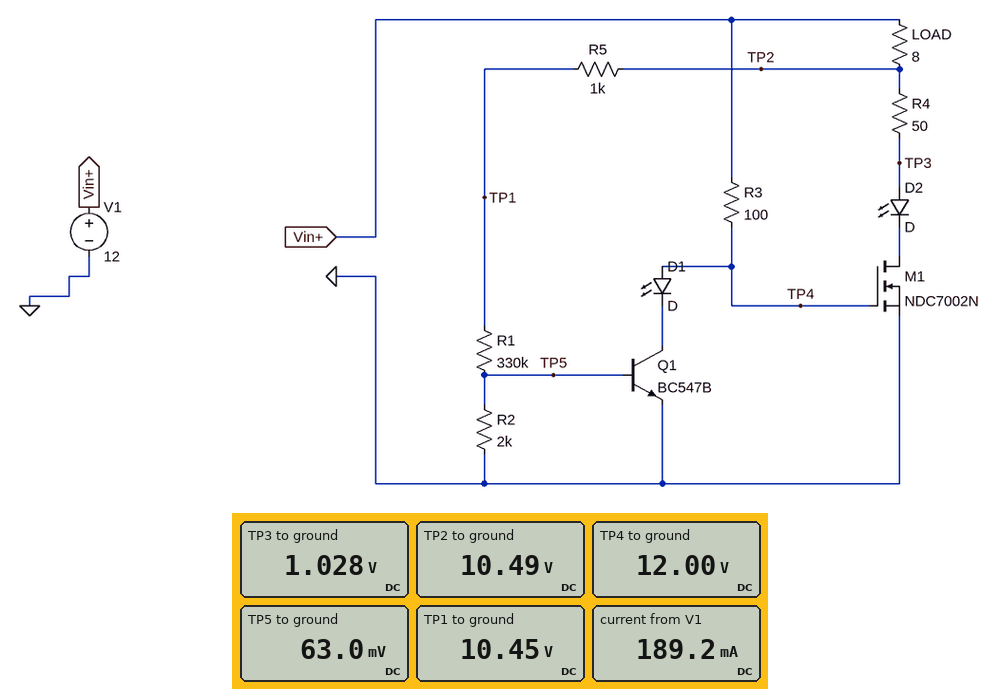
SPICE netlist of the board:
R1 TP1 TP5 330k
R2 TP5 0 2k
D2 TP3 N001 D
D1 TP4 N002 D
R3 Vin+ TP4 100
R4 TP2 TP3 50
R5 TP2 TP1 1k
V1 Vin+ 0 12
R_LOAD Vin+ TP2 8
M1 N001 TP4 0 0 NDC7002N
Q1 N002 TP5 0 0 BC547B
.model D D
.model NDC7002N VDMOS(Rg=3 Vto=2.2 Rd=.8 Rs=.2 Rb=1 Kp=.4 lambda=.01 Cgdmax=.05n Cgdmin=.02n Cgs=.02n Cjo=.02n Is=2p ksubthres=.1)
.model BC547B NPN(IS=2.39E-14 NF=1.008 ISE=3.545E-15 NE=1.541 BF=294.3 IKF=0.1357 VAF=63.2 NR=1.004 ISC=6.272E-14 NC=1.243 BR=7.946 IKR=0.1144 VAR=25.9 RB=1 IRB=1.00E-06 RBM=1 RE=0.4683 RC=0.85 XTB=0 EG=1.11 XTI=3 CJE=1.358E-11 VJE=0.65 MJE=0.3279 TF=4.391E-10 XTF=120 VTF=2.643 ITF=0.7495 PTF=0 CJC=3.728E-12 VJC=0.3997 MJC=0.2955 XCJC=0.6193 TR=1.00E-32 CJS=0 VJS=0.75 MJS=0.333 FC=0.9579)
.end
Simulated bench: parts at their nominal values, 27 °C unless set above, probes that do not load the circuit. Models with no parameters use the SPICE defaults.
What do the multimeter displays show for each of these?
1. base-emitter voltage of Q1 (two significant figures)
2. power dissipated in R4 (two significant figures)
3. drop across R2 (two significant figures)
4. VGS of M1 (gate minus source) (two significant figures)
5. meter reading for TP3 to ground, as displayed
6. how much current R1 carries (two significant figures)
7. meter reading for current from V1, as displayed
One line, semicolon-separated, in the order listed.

63 mV; 1.8 W; 63 mV; 12 V; 1.028 V; 31 µA; 189.2 mA
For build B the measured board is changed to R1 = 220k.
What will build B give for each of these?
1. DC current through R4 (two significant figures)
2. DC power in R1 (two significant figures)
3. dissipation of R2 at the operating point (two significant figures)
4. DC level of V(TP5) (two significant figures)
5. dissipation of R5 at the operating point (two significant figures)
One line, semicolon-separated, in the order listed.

190 mA; 490 µW; 4.4 µW; 94 mV; 2.2 µW
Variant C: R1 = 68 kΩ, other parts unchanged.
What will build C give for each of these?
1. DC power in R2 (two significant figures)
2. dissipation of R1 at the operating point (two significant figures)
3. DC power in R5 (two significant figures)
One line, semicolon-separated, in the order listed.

44 µW; 1.5 mW; 22 µW
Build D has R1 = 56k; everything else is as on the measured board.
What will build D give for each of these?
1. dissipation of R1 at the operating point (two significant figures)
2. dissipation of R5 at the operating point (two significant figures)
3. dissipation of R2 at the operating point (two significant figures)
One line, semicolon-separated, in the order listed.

1.8 mW; 32 µW; 63 µW
